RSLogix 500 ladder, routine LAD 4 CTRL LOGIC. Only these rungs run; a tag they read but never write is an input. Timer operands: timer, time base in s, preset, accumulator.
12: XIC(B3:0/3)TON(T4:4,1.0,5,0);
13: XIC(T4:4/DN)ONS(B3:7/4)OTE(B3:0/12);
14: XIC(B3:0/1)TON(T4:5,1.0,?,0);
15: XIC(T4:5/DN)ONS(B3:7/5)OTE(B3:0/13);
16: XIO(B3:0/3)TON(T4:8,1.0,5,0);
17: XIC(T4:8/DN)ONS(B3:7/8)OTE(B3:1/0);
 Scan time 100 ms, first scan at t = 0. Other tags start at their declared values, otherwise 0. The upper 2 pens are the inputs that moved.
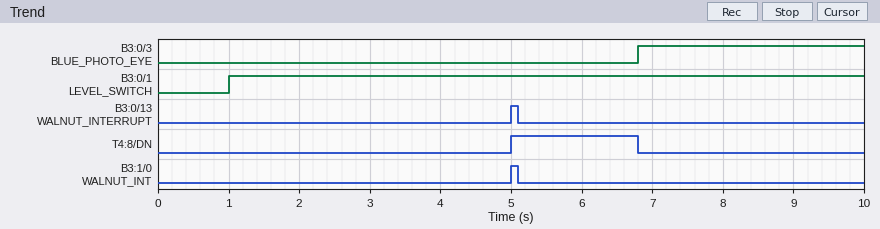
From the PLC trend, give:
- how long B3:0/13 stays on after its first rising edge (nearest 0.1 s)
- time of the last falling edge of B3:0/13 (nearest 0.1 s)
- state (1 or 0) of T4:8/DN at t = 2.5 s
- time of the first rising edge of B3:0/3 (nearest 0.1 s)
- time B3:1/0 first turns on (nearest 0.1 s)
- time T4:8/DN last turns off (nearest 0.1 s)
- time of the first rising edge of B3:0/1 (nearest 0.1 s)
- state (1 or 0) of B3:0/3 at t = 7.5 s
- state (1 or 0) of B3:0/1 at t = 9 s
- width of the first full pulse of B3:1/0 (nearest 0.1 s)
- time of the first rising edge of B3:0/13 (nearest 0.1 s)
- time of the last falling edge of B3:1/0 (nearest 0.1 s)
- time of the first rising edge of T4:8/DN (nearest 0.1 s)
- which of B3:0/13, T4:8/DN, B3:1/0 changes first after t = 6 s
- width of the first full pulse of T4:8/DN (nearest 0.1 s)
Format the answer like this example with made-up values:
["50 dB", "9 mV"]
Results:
["0.1 s", "5.1 s", "0", "6.8 s", "5.0 s", "6.8 s", "1.0 s", "1", "1", "0.1 s", "5.0 s", "5.1 s", "5.0 s", "T4:8/DN", "1.8 s"]
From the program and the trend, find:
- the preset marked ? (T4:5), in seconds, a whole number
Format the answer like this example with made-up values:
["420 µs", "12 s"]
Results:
["4 s"]
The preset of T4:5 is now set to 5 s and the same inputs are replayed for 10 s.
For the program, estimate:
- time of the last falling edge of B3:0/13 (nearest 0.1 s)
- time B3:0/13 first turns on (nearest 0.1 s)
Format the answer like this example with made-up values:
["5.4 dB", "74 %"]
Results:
["6.1 s", "6.0 s"]
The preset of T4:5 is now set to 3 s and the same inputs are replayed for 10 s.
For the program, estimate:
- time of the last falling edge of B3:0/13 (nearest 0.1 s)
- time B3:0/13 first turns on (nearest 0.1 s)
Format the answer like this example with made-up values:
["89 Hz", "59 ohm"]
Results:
["4.1 s", "4.0 s"]
